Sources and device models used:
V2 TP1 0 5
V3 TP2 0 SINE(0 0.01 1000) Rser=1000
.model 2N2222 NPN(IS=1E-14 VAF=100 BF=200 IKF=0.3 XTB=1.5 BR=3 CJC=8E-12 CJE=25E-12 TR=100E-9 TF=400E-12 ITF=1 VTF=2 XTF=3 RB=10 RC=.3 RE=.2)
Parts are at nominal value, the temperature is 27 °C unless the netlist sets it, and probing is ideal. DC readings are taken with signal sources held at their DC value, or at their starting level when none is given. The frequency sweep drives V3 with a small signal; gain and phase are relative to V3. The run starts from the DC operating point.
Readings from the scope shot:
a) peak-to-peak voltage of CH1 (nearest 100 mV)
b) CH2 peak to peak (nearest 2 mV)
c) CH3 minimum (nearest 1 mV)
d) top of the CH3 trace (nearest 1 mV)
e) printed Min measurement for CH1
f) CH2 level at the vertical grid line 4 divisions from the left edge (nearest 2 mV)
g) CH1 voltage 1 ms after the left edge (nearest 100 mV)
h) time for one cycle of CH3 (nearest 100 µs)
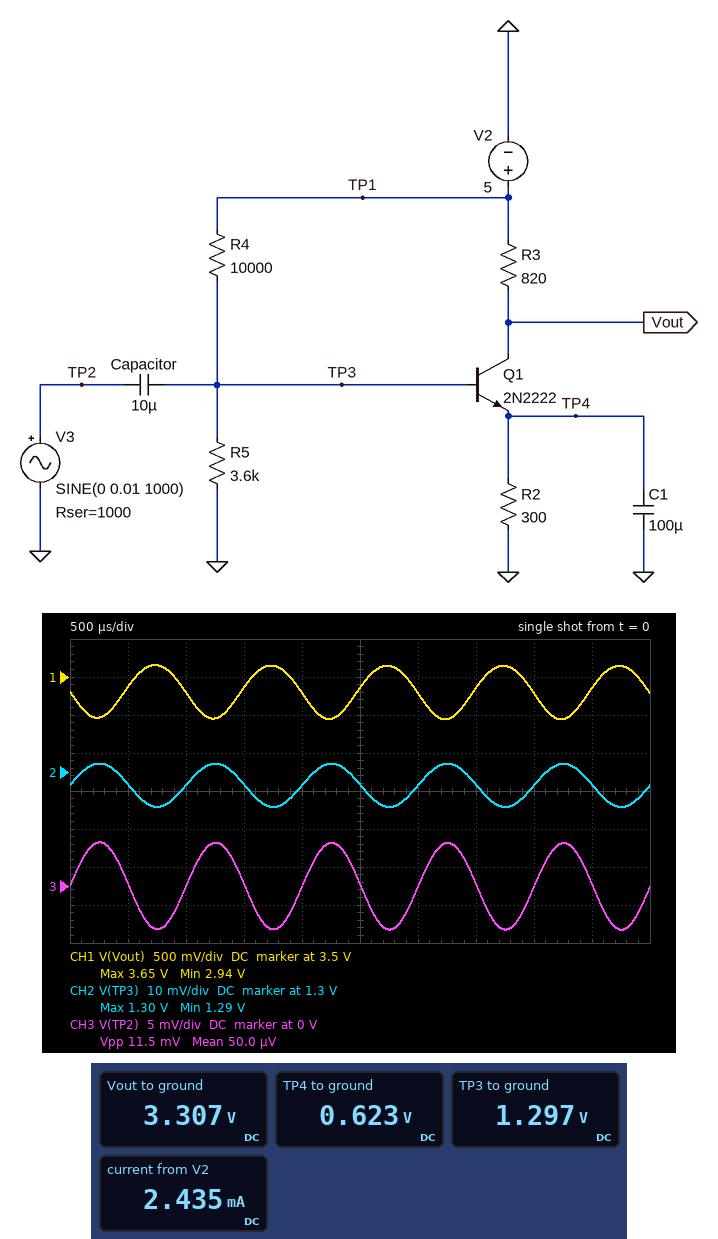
700 mV
12 mV
-6 mV
6 mV
2.94 V
1.296 V
3.3 V
1.0 ms
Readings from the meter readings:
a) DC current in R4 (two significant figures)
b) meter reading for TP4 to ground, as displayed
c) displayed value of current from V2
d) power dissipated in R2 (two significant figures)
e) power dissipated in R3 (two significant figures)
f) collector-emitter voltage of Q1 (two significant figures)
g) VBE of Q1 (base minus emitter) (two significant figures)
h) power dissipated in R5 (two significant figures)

370 µA
0.623 V
2.435 mA
1.3 mW
3.5 mW
2.7 V
670 mV
470 µW
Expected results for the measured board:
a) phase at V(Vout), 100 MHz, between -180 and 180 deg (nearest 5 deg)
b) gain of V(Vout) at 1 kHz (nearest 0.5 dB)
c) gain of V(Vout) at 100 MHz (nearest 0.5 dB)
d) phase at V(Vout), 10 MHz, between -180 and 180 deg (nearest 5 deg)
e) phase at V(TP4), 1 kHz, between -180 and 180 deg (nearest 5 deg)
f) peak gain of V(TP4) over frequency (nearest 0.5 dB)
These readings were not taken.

65 deg
31.0 dB
-13.0 dB
90 deg
-85 deg
-4.0 dB
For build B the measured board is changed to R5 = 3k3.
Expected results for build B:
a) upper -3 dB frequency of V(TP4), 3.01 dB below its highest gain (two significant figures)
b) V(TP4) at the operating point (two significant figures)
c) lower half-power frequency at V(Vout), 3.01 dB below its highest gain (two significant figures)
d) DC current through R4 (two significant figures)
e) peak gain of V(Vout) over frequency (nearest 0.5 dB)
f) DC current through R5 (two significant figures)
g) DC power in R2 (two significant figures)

100 Hz
550 mV
95 Hz
380 µA
30.0 dB
370 µA
1.0 mW
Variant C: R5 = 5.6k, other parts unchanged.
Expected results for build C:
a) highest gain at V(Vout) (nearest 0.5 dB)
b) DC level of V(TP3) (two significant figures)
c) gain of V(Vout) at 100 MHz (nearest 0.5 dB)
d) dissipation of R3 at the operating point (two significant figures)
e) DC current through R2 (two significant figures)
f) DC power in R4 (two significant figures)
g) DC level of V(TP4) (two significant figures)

34.5 dB
1.7 V
-14.5 dB
9.8 mW
3.5 mA
1.1 mW
1.0 V
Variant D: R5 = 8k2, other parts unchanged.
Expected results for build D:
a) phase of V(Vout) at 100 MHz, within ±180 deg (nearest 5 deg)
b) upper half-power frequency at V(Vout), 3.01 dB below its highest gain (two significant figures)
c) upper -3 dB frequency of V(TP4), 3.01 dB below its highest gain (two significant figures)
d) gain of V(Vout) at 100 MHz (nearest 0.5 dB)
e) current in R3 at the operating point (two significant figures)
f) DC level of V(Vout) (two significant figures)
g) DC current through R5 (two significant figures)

15 deg
530 kHz
30 Hz
-43.5 dB
4.4 mA
1.4 V
250 µA
